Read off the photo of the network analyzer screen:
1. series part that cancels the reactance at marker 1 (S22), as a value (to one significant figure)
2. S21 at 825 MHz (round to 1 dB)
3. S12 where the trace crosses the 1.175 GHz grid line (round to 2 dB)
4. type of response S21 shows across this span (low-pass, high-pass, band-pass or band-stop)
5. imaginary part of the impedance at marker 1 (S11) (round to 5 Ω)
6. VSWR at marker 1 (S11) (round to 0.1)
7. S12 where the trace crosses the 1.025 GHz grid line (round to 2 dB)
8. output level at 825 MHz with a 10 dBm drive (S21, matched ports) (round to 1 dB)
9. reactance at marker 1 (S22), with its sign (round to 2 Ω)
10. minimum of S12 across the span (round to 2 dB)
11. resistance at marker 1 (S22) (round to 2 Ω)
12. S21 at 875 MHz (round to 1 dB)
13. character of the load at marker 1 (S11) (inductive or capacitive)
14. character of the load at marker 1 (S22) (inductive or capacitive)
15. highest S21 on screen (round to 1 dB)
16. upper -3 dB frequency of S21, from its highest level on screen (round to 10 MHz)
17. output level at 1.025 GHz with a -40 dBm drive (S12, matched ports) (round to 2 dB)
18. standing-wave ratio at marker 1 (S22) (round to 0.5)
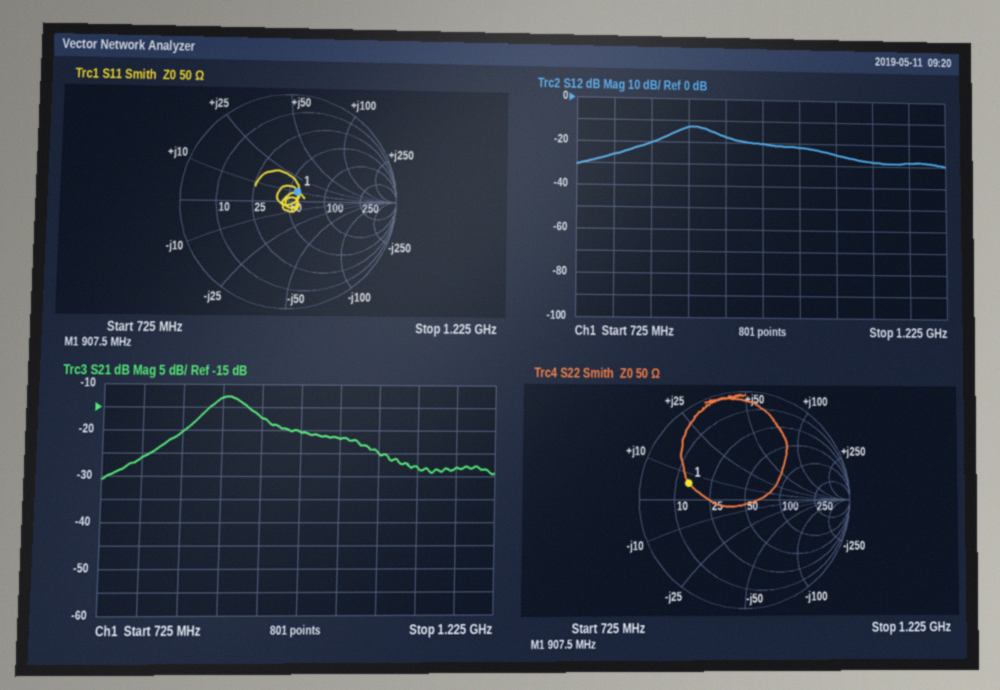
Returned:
30 pF
-20 dB
-28 dB
band-pass
+10 Ω
1.3
-22 dB
-10 dBm
+6 Ω
-30 dB
14 Ω
-13 dB
inductive
inductive
-13 dB
910 MHz
-62 dBm
3.5
